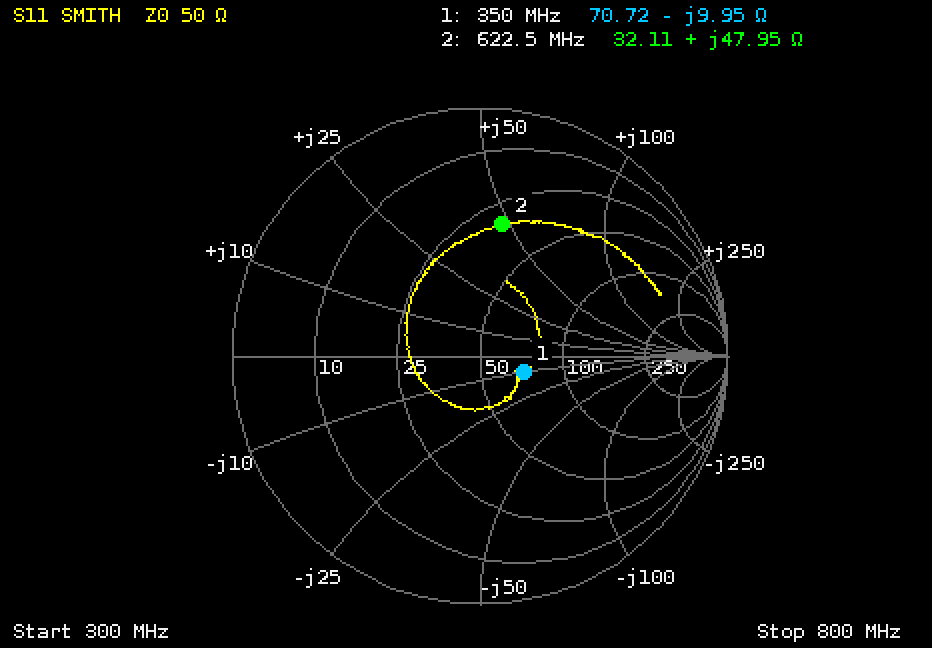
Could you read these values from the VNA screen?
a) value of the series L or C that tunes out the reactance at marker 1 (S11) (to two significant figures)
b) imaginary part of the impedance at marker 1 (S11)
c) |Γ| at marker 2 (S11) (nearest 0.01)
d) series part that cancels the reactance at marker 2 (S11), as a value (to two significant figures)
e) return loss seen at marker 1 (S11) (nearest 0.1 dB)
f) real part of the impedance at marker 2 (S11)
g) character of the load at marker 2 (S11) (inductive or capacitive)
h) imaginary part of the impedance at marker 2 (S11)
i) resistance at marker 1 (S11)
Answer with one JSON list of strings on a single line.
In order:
["4.5 nH", "-9.95 Ω", "0.54", "5.3 pF", "14.4 dB", "32.11 Ω", "inductive", "+47.95 Ω", "70.72 Ω"]
